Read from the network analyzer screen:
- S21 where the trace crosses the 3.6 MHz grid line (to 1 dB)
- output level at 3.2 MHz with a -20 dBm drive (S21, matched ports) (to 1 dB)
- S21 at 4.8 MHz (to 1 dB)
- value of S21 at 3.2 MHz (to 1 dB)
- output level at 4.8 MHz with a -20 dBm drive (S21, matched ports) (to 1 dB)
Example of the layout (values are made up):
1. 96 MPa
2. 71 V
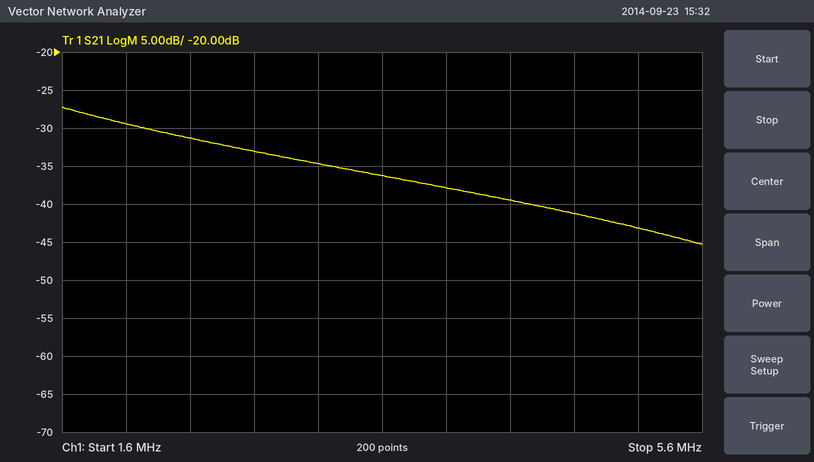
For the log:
1. -36 dB
2. -55 dBm
3. -41 dB
4. -35 dB
5. -61 dBm
